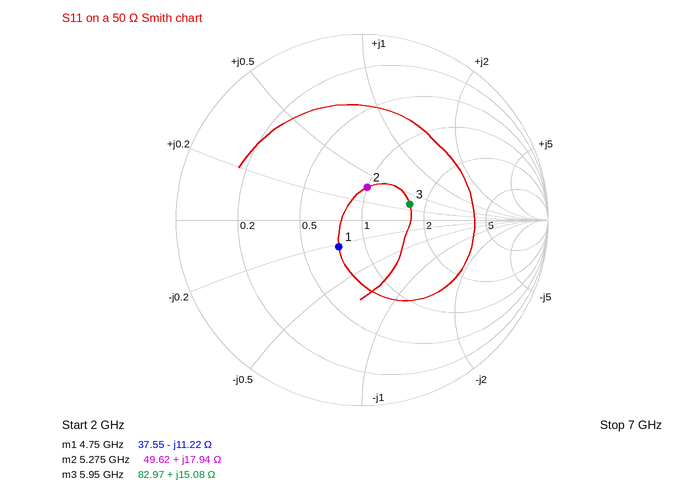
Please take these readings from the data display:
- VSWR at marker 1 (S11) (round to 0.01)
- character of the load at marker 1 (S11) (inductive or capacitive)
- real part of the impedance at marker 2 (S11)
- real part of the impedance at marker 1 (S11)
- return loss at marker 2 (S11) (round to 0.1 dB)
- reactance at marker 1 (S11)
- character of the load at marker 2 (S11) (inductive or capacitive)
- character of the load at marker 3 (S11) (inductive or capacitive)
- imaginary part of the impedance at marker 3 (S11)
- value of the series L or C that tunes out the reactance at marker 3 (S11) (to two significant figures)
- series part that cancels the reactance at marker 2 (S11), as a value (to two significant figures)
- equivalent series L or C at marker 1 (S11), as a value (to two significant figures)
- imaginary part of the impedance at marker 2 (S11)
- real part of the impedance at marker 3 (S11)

1.47
capacitive
49.62 Ω
37.55 Ω
15.0 dB
-11.22 Ω
inductive
inductive
+15.08 Ω
1.8 pF
1.7 pF
3.0 pF
+17.94 Ω
82.97 Ω
